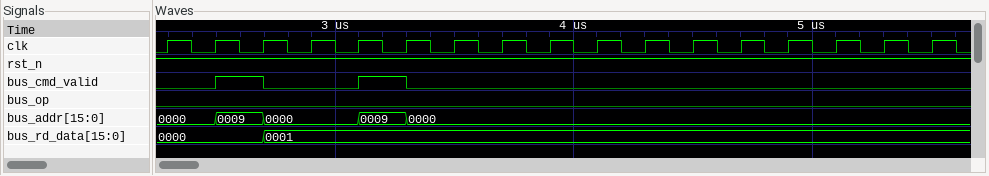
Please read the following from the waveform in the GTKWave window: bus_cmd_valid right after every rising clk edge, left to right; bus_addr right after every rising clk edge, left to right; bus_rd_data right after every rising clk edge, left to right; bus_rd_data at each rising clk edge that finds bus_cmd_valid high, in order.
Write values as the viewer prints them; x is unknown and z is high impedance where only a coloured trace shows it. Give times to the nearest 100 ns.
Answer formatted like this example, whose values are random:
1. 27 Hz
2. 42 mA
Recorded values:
1. 0 1 0 0 1 0 0 0 0 0 0 0 0 0 0 0 0
2. 0000, 0009, 0000, 0000, 0009, 0000, 0000, 0000, 0000, 0000, 0000, 0000, 0000, 0000, 0000, 0000, 0000
3. 0000, 0000, 0001, 0001, 0001, 0001, 0001, 0001, 0001, 0001, 0001, 0001, 0001, 0001, 0001, 0001, 0001
4. 0000, 0001
